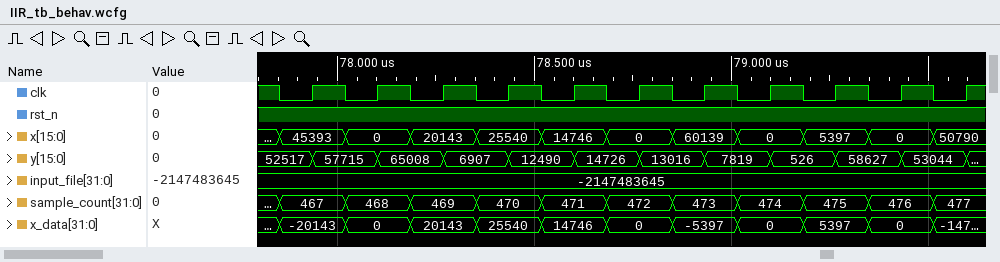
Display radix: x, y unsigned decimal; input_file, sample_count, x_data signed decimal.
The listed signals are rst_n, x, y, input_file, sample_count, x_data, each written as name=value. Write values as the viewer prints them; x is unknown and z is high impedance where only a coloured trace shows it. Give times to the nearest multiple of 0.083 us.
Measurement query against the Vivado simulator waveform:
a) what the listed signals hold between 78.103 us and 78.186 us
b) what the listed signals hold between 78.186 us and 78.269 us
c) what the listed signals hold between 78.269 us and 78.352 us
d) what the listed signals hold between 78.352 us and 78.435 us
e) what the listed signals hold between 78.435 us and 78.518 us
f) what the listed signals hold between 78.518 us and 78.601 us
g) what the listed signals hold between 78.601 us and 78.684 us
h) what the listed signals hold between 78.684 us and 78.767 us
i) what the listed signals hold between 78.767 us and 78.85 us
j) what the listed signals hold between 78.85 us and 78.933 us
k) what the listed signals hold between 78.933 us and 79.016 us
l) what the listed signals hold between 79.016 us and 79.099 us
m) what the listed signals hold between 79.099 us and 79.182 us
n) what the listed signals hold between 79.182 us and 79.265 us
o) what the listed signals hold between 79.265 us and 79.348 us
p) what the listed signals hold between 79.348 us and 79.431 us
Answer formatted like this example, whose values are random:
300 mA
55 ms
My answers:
rst_n=1, x=0, y=65008, input_file=-2147483645, sample_count=468, x_data=0
rst_n=1, x=20143, y=65008, input_file=-2147483645, sample_count=469, x_data=20143
rst_n=1, x=20143, y=6907, input_file=-2147483645, sample_count=469, x_data=20143
rst_n=1, x=25540, y=6907, input_file=-2147483645, sample_count=470, x_data=25540
rst_n=1, x=25540, y=12490, input_file=-2147483645, sample_count=470, x_data=25540
rst_n=1, x=14746, y=12490, input_file=-2147483645, sample_count=471, x_data=14746
rst_n=1, x=14746, y=14726, input_file=-2147483645, sample_count=471, x_data=14746
rst_n=1, x=0, y=14726, input_file=-2147483645, sample_count=472, x_data=0
rst_n=1, x=0, y=13016, input_file=-2147483645, sample_count=472, x_data=0
rst_n=1, x=60139, y=13016, input_file=-2147483645, sample_count=473, x_data=-5397
rst_n=1, x=60139, y=7819, input_file=-2147483645, sample_count=473, x_data=-5397
rst_n=1, x=0, y=7819, input_file=-2147483645, sample_count=474, x_data=0
rst_n=1, x=0, y=526, input_file=-2147483645, sample_count=474, x_data=0
rst_n=1, x=5397, y=526, input_file=-2147483645, sample_count=475, x_data=5397
rst_n=1, x=5397, y=58627, input_file=-2147483645, sample_count=475, x_data=5397
rst_n=1, x=0, y=58627, input_file=-2147483645, sample_count=476, x_data=0
